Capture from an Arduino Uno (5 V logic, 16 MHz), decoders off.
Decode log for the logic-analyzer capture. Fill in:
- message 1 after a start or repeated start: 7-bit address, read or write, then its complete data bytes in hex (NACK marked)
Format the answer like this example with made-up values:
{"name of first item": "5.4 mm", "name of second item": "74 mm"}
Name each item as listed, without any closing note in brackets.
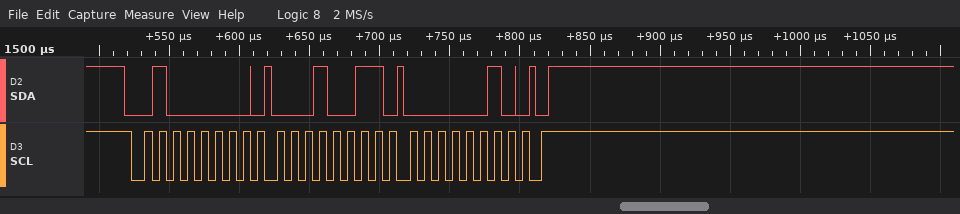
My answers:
{"message 1 after a start or repeated start: 7-bit address, read or write, then its complete data bytes in hex": "0x20 write: 13 02"}
